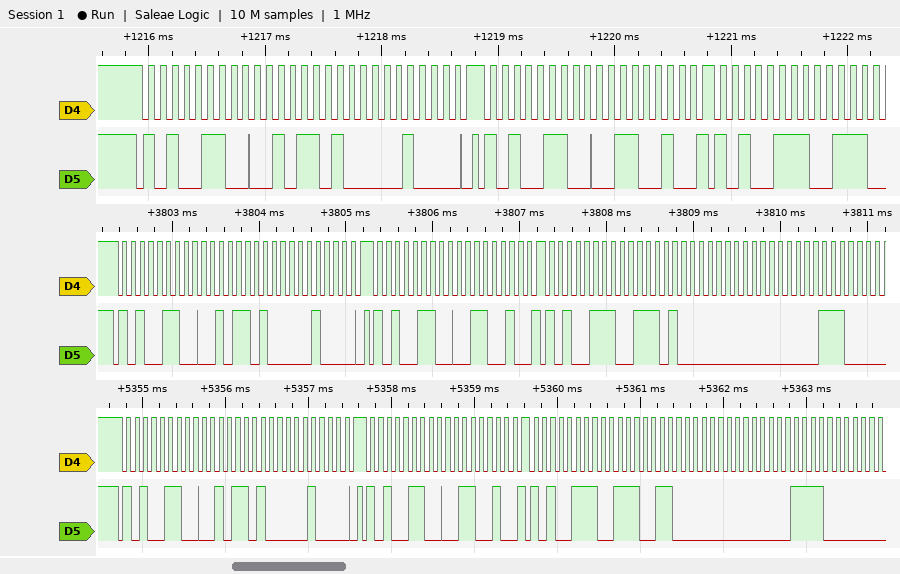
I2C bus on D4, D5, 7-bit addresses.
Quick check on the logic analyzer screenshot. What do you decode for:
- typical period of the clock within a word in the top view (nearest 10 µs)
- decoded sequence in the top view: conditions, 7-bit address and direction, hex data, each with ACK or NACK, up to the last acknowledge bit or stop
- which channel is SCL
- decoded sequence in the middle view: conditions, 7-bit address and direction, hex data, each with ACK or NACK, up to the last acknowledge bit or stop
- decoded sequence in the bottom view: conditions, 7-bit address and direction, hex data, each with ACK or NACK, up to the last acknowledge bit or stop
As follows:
100 µs
start, address 53 write ACK, 2D ACK, 08 ACK, stop, start, address 53 write ACK, 32 ACK, repeated start, address 53 read ACK
D4
start, address 53 write ACK, 2D ACK, 08 ACK, stop, start, address 53 write ACK, 32 ACK, repeated start, address 53 read ACK, 74 ACK, 00 ACK, 0E ACK
start, address 53 write ACK, 2D ACK, 08 ACK, stop, start, address 53 write ACK, 32 ACK, repeated start, address 53 read ACK, 73 ACK, 00 ACK, 0F ACK
